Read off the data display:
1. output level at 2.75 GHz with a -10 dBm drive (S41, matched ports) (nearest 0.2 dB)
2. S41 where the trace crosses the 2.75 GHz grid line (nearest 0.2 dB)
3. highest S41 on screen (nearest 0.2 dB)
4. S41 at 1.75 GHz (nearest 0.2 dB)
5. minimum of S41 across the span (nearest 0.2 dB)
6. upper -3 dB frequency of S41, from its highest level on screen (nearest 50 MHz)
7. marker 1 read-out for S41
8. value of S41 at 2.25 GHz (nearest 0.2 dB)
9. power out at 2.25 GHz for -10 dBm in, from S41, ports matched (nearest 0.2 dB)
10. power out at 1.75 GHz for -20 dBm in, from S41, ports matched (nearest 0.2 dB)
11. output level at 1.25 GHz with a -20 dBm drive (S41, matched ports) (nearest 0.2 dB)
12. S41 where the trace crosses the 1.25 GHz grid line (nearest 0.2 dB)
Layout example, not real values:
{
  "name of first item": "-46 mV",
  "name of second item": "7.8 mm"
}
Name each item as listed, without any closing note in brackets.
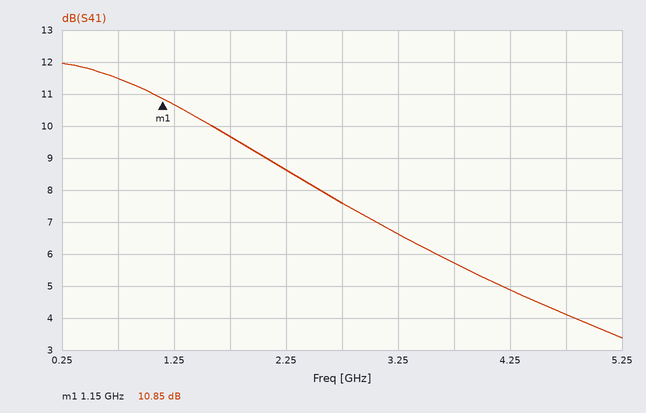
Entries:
{
  "output level at 2.75 GHz with a -10 dBm drive (S41, matched ports)": "-2.4 dBm",
  "S41 where the trace crosses the 2.75 GHz grid line": "7.6 dB",
  "highest S41 on screen": "12.0 dB",
  "S41 at 1.75 GHz": "9.6 dB",
  "minimum of S41 across the span": "3.4 dB",
  "upper -3 dB frequency of S41, from its highest level on screen": "2.10 GHz",
  "marker 1 read-out for S41": "10.85 dB",
  "value of S41 at 2.25 GHz": "8.6 dB",
  "power out at 2.25 GHz for -10 dBm in, from S41, ports matched": "-1.4 dBm",
  "power out at 1.75 GHz for -20 dBm in, from S41, ports matched": "-10.4 dBm",
  "output level at 1.25 GHz with a -20 dBm drive (S41, matched ports)": "-9.4 dBm",
  "S41 where the trace crosses the 1.25 GHz grid line": "10.6 dB"
}
